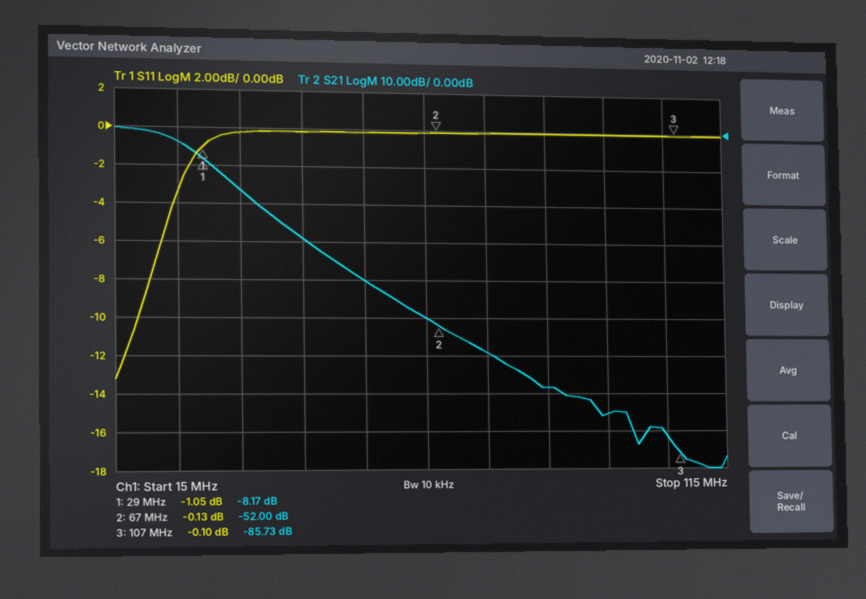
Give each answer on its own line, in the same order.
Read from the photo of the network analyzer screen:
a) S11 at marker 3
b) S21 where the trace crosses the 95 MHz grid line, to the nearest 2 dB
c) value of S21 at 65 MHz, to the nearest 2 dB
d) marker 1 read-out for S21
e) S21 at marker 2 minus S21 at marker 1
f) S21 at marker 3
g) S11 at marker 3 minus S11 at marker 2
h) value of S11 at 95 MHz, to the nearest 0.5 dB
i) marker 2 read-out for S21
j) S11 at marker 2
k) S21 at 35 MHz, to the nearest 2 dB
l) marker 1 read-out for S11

-0.10 dB
-76 dB
-50 dB
-8.17 dB
-43.83 dB
-85.73 dB
0.03 dB
0.0 dB
-52.00 dB
-0.13 dB
-16 dB
-1.05 dB
